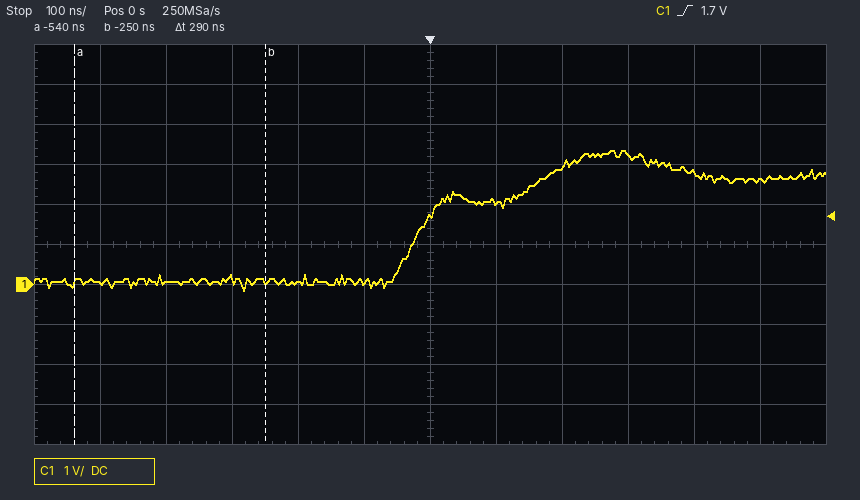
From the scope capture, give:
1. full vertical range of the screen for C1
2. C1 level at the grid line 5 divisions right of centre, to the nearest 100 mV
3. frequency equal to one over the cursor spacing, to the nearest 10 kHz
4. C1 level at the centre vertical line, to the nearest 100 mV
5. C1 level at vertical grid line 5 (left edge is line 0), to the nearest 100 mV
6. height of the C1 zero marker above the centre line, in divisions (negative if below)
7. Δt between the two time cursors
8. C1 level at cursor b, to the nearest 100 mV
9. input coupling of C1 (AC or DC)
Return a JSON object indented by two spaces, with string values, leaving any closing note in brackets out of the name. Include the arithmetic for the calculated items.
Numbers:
{
  "full vertical range of the screen for C1": "10 V",
  "C1 level at the grid line 5 divisions right of centre, to the nearest 100 mV": "2.6 V",
  "frequency equal to one over the cursor spacing, to the nearest 10 kHz": "1 / 290 ns ≈ 3.45 MHz",
  "C1 level at the centre vertical line, to the nearest 100 mV": "1.7 V",
  "C1 level at vertical grid line 5 (left edge is line 0), to the nearest 100 mV": "100 mV",
  "height of the C1 zero marker above the centre line, in divisions": "-1.0 div",
  "Δt between the two time cursors": "290 ns",
  "C1 level at cursor b, to the nearest 100 mV": "100 mV",
  "input coupling of C1": "DC"
}
